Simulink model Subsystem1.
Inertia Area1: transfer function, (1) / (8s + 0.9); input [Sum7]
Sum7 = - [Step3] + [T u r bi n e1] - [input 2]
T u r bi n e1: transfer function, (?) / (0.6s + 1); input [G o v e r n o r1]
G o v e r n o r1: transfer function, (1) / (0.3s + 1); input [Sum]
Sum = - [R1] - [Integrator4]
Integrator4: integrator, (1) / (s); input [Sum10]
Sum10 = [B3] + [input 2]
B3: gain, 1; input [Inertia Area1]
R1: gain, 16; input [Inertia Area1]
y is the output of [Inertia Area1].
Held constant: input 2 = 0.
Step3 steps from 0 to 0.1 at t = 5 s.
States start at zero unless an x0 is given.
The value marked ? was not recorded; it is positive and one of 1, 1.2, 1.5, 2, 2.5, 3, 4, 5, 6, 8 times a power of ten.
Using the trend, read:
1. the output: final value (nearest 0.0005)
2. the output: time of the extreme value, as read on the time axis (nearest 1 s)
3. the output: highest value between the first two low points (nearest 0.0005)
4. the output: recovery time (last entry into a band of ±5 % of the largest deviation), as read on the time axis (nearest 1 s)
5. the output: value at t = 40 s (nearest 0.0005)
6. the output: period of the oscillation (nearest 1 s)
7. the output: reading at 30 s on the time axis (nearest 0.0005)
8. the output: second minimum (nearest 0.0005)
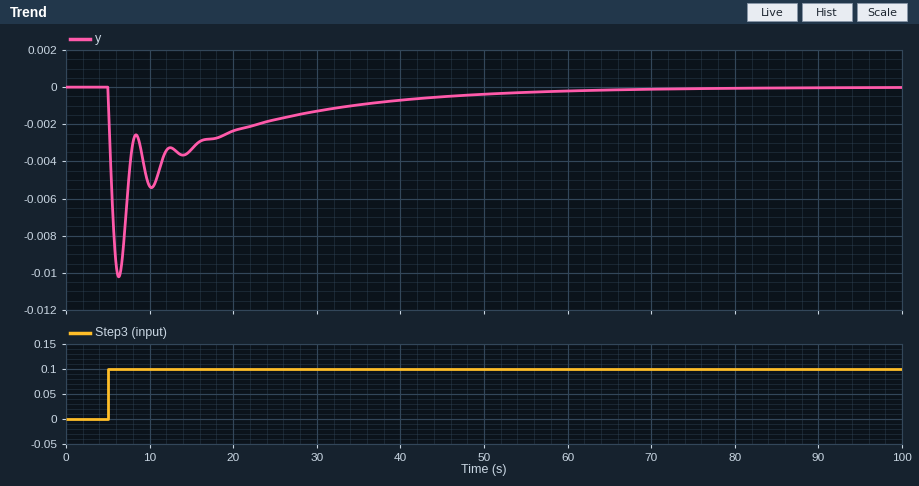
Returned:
0.0000
6 s
-0.0025
45 s
-0.0005
4 s
-0.0015
-0.0055
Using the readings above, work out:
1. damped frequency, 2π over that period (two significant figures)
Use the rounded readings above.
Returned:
1.6 rad/s
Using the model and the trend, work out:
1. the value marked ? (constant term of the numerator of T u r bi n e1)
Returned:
1
